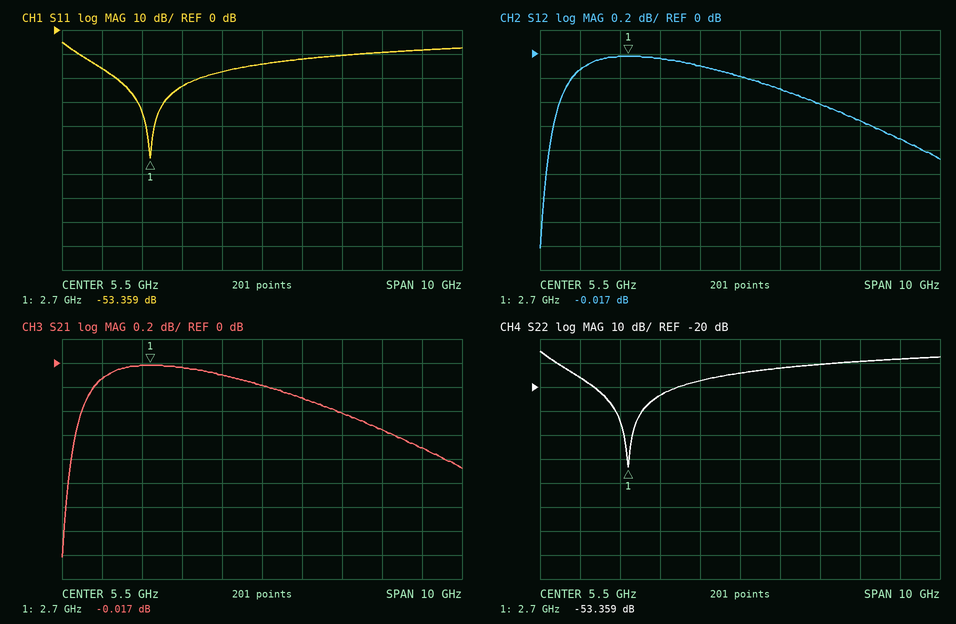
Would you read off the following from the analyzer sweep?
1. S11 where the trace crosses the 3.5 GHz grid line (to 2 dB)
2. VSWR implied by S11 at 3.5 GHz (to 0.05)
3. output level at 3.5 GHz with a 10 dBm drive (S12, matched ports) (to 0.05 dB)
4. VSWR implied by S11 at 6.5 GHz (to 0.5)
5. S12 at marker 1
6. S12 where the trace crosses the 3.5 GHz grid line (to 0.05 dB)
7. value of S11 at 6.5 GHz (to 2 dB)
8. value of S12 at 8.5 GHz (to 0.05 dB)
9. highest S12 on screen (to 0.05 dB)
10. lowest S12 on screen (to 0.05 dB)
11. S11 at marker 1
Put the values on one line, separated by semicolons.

-24 dB; 1.15; 9.95 dBm; 1.5; -0.017 dB; -0.05 dB; -12 dB; -0.55 dB; 0.00 dB; -1.60 dB; -53.359 dB
